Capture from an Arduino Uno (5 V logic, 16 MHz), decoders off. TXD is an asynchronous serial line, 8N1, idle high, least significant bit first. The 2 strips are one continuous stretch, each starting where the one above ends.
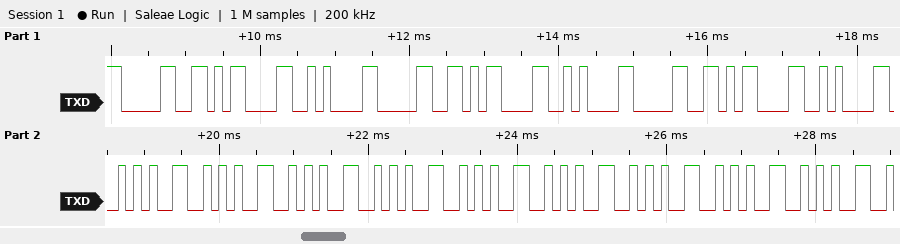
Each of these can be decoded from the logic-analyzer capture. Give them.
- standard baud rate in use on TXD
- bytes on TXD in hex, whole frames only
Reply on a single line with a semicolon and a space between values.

9600 baud; 0x30 0x0D 0x0A 0x30 0x0D 0x0A 0x30 0x0D 0x0A 0x2A 0x2A 0x2A 0x2A 0x2A 0x2A 0x2A 0x2A 0x2A
